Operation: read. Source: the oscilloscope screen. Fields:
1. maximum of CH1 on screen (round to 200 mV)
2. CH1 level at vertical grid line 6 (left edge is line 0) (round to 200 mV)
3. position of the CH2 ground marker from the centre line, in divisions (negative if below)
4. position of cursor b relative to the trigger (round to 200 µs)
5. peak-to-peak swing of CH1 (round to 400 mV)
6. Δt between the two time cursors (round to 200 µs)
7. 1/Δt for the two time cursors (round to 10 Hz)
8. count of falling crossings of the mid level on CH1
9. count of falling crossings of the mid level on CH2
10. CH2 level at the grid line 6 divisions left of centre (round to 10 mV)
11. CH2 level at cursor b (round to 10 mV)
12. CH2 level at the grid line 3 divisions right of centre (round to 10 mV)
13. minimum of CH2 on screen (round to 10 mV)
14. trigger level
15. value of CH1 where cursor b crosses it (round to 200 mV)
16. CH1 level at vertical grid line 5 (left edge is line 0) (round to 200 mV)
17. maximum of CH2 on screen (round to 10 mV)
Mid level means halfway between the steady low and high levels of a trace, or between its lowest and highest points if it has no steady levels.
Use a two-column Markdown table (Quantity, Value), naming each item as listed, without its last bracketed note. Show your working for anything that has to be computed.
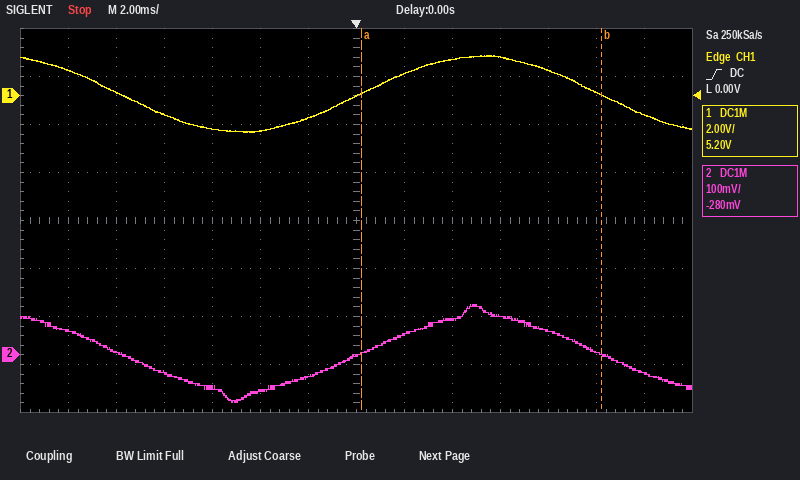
| Quantity | Value |
|---|---|
| maximum of CH1 on screen | 1.6 V |
| CH1 level at vertical grid line 6 (left edge is line 0) | -1.0 V |
| position of the CH2 ground marker from the centre line, in divisions | -2.8 div |
| position of cursor b relative to the trigger | +10.2 ms |
| peak-to-peak swing of CH1 | 3.2 V |
| Δt between the two time cursors | 10.0 ms |
| 1/Δt for the two time cursors | 1 / 10.0 ms ≈ 100 Hz |
| count of falling crossings of the mid level on CH1 | 2 |
| count of falling crossings of the mid level on CH2 | 2 |
| CH2 level at the grid line 6 divisions left of centre | 50 mV |
| CH2 level at cursor b | 0 mV |
| CH2 level at the grid line 3 divisions right of centre | 80 mV |
| minimum of CH2 on screen | -100 mV |
| trigger level | 0.00 V |
| value of CH1 where cursor b crosses it | 0.0 V |
| CH1 level at vertical grid line 5 (left edge is line 0) | -1.4 V |
| maximum of CH2 on screen | 100 mV |
